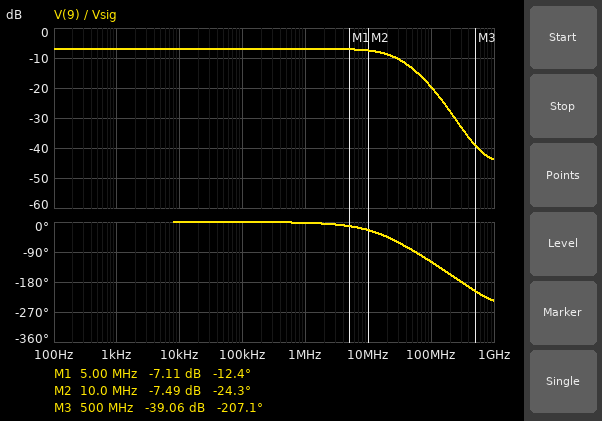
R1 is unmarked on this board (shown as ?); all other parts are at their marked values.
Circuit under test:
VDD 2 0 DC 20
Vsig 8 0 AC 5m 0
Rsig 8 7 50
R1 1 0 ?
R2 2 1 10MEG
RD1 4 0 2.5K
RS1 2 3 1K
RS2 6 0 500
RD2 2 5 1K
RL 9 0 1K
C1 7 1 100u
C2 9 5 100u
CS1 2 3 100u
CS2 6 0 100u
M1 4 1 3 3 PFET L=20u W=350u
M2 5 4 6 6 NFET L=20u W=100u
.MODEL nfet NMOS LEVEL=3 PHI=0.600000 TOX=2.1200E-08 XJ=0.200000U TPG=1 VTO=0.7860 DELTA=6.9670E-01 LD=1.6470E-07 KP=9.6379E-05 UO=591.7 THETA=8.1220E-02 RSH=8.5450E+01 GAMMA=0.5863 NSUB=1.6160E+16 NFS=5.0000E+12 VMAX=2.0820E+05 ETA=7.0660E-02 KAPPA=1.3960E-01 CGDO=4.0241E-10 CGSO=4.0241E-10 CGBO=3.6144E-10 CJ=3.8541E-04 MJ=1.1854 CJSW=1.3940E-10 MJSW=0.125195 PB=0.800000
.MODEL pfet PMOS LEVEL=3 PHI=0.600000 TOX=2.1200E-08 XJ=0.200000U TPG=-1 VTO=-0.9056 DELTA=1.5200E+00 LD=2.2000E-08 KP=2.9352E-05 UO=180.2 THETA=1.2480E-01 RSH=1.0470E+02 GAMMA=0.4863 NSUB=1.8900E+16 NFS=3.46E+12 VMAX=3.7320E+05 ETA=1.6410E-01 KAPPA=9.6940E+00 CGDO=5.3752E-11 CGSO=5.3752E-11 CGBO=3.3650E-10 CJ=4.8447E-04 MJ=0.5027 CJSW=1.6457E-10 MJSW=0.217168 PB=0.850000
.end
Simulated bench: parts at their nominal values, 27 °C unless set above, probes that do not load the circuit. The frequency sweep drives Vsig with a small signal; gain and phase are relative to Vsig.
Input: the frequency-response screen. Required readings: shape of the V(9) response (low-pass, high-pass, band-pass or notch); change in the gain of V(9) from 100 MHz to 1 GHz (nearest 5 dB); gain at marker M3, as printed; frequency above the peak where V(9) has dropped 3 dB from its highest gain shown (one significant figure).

low-pass
-25 dB
-39.06 dB
30 MHz
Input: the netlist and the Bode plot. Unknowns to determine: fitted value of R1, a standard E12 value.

33 MΩ
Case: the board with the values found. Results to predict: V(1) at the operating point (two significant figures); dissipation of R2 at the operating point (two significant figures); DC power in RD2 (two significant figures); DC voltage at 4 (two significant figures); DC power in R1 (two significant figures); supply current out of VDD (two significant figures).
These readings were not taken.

15 V
2.2 µW
230 µW
2.7 V
7.1 µW
1.6 mA
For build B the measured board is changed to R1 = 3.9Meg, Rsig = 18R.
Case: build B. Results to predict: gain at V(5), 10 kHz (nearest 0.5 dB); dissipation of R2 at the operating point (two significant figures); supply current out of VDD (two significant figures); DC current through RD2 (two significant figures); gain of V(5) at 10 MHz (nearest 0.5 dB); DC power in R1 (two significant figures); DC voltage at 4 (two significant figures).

-17.0 dB
21 µW
11 mA
6.3 mA
-14.0 dB
8.1 µW
12 V
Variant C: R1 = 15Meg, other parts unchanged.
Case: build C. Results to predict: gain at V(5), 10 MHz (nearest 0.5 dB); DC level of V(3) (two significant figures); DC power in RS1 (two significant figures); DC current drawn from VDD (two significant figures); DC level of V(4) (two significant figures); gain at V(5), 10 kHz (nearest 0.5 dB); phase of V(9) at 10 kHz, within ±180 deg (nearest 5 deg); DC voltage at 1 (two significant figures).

0.5 dB
17 V
6.7 mW
5.2 mA
6.5 V
1.0 dB
0 deg
12 V
